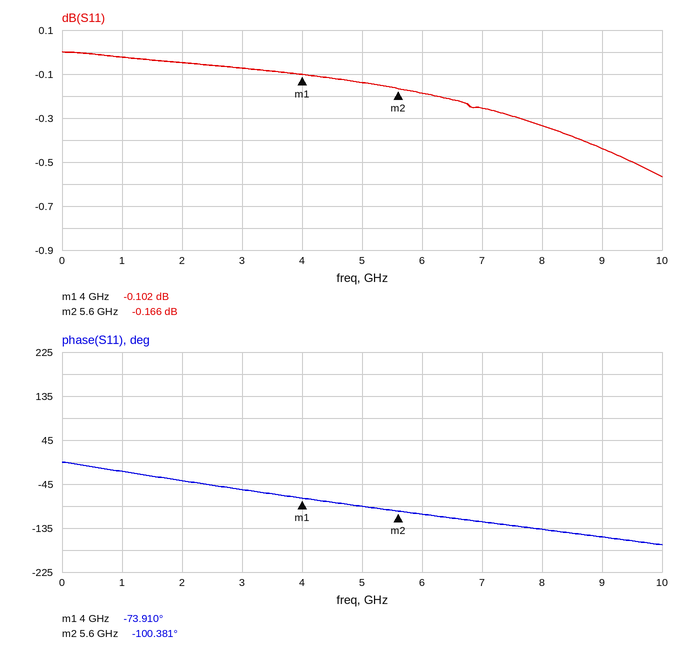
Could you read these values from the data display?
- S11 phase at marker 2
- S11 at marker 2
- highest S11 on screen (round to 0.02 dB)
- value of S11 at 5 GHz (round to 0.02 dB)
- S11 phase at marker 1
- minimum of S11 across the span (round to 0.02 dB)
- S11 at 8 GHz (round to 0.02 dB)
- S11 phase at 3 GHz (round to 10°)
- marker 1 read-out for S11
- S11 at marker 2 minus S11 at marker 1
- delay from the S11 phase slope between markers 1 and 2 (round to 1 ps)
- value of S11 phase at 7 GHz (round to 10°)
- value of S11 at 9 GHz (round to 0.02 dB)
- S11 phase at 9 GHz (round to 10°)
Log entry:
-100.381°
-0.166 dB
0.00 dB
-0.14 dB
-73.910°
-0.56 dB
-0.34 dB
-60°
-0.102 dB
-0.064 dB
46 ps
-120°
-0.44 dB
-150°
